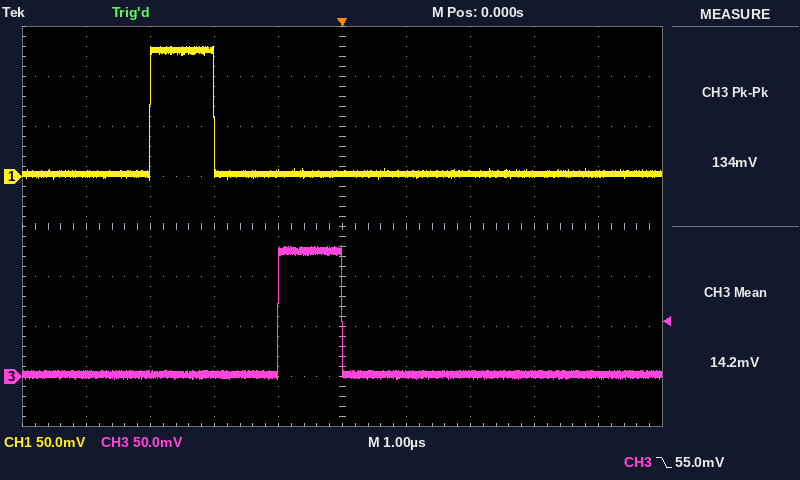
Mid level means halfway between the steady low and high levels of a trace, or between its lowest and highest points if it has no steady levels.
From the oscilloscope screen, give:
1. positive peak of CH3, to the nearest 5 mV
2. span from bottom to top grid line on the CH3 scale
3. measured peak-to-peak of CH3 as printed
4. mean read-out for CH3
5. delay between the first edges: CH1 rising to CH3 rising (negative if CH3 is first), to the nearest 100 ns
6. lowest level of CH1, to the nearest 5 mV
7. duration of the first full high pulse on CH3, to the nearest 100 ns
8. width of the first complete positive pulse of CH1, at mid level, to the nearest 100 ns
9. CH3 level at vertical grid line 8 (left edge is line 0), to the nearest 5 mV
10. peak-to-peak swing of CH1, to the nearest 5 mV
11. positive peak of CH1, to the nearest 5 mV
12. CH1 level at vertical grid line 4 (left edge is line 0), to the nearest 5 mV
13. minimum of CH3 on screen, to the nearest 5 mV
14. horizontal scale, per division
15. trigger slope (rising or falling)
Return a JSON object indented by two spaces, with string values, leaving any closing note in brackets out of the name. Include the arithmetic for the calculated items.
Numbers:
{
  "positive peak of CH3, to the nearest 5 mV": "130 mV",
  "span from bottom to top grid line on the CH3 scale": "400 mV",
  "measured peak-to-peak of CH3 as printed": "134 mV",
  "mean read-out for CH3": "14.2 mV",
  "delay between the first edges: CH1 rising to CH3 rising (negative if CH3 is first), to the nearest 100 ns": "+2.0 µs",
  "lowest level of CH1, to the nearest 5 mV": "-5 mV",
  "duration of the first full high pulse on CH3, to the nearest 100 ns": "1.0 µs",
  "width of the first complete positive pulse of CH1, at mid level, to the nearest 100 ns": "1.0 µs",
  "CH3 level at vertical grid line 8 (left edge is line 0), to the nearest 5 mV": "0 mV",
  "peak-to-peak swing of CH1, to the nearest 5 mV": "130 mV − (-5 mV) = 135 mV",
  "positive peak of CH1, to the nearest 5 mV": "130 mV",
  "CH1 level at vertical grid line 4 (left edge is line 0), to the nearest 5 mV": "5 mV",
  "minimum of CH3 on screen, to the nearest 5 mV": "-5 mV",
  "horizontal scale, per division": "1 µs",
  "trigger slope": "falling"
}
